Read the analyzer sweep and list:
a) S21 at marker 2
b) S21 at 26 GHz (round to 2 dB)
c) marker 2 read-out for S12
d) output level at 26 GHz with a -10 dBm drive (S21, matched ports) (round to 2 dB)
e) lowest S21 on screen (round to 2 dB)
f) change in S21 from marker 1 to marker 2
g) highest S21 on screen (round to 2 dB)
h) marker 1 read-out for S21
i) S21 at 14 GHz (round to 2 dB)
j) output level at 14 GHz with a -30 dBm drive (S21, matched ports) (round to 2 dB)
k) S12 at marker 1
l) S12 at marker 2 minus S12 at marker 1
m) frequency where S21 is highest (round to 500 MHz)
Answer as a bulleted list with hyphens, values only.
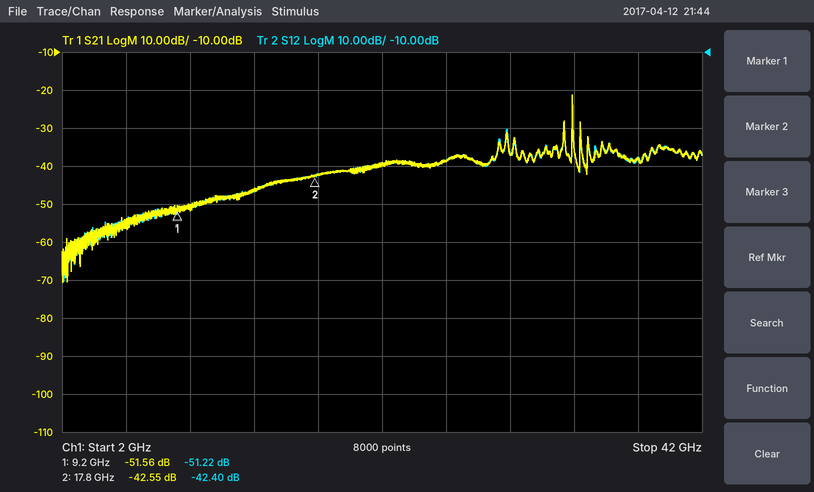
- -42.55 dB
- -38 dB
- -42.40 dB
- -48 dBm
- -70 dB
- 9.01 dB
- -22 dB
- -51.56 dB
- -46 dB
- -76 dBm
- -51.22 dB
- 8.82 dB
- 34.0 GHz
